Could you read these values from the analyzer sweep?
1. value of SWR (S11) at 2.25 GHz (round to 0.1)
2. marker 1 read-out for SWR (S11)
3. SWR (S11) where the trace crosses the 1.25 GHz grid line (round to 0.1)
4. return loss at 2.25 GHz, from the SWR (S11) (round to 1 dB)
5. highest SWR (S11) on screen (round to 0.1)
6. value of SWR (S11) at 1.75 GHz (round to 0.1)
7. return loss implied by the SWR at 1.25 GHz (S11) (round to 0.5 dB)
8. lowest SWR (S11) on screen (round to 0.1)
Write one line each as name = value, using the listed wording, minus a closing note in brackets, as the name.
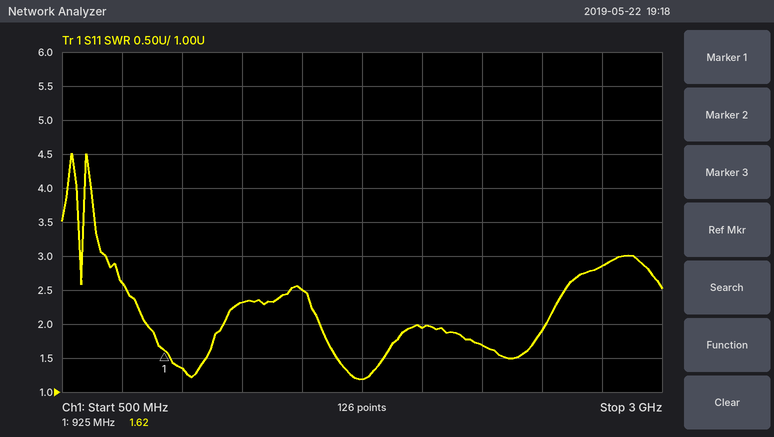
value of SWR (S11) at 2.25 GHz = 1.7
marker 1 read-out for SWR = 1.62
SWR (S11) where the trace crosses the 1.25 GHz grid line = 2.3
return loss at 2.25 GHz, from the SWR (S11) = 12 dB
highest SWR (S11) on screen = 4.5
value of SWR (S11) at 1.75 GHz = 1.2
return loss implied by the SWR at 1.25 GHz (S11) = 8.0 dB
lowest SWR (S11) on screen = 1.2
